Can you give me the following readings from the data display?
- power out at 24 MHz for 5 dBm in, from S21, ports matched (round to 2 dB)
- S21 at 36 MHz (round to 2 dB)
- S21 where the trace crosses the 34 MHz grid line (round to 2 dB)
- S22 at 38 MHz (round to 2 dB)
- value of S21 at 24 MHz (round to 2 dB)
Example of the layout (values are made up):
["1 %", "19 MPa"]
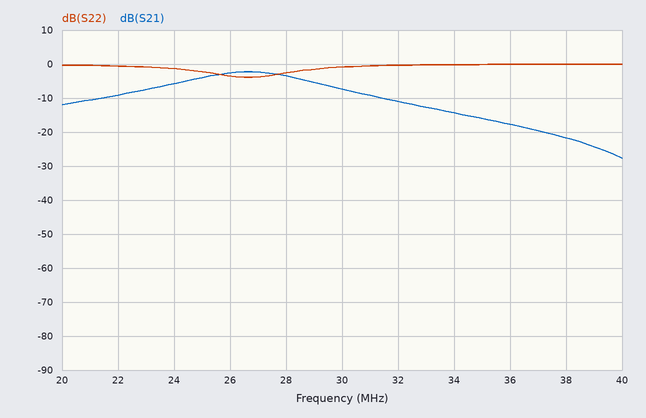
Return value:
["0 dBm", "-18 dB", "-14 dB", "0 dB", "-6 dB"]
